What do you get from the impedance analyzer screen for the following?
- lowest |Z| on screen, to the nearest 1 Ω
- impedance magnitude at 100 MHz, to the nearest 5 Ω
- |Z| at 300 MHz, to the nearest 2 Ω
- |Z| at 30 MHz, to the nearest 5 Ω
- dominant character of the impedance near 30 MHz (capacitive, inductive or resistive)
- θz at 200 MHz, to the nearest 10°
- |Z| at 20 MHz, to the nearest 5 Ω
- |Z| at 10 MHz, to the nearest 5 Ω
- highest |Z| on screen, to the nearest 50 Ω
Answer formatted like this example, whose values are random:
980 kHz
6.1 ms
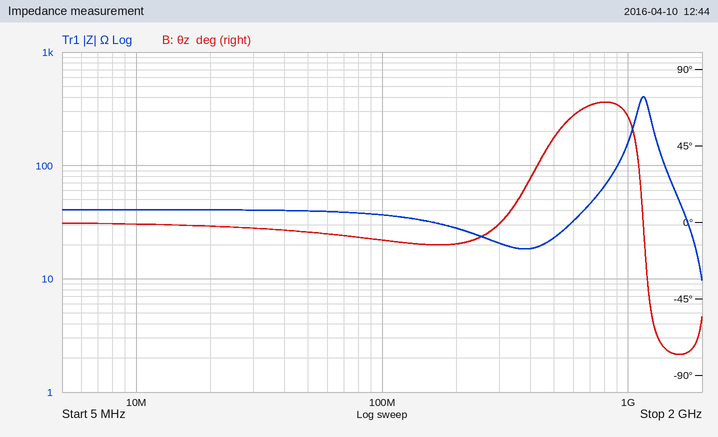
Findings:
10 Ω
35 Ω
20 Ω
40 Ω
resistive
-10°
40 Ω
40 Ω
400 Ω
